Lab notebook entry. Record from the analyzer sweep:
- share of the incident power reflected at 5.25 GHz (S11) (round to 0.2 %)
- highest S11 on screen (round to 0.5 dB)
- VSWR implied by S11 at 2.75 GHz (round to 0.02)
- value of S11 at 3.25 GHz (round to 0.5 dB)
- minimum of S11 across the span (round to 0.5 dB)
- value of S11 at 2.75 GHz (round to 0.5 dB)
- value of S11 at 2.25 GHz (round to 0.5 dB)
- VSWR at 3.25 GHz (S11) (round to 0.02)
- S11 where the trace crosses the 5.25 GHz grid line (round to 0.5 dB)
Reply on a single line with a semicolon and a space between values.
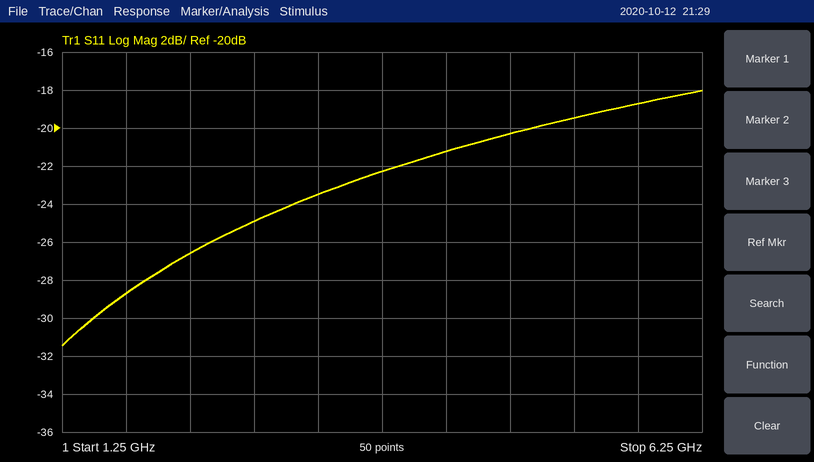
1.2 %; -18.0 dB; 1.12; -23.5 dB; -31.5 dB; -25.0 dB; -26.5 dB; 1.14; -19.5 dB
